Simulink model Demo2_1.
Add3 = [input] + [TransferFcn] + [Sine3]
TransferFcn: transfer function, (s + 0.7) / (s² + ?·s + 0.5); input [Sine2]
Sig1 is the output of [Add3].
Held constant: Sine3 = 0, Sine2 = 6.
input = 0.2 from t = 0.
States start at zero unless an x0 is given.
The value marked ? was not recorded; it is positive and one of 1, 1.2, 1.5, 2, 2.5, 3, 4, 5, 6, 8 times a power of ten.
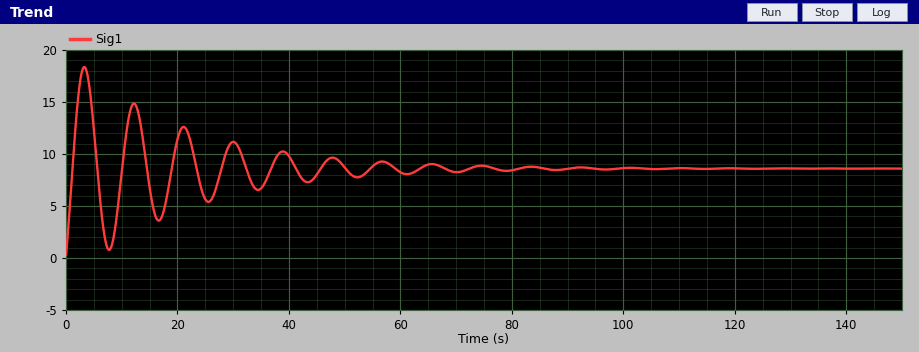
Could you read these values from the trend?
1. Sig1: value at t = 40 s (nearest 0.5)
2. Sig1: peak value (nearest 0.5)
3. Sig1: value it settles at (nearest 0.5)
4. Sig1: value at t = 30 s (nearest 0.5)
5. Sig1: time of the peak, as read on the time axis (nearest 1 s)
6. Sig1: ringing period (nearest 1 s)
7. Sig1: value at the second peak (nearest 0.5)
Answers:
10.0
18.5
8.5
11.0
3 s
9 s
15.0
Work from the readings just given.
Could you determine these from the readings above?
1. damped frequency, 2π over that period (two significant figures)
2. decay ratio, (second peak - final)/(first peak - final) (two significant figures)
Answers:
0.70 rad/s
0.65
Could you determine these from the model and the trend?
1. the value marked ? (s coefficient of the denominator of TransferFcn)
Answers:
0.1
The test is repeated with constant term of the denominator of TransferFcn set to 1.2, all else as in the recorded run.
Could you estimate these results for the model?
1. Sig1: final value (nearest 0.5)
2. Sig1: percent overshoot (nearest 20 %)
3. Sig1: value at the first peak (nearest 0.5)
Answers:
3.5
160 %
9.5
